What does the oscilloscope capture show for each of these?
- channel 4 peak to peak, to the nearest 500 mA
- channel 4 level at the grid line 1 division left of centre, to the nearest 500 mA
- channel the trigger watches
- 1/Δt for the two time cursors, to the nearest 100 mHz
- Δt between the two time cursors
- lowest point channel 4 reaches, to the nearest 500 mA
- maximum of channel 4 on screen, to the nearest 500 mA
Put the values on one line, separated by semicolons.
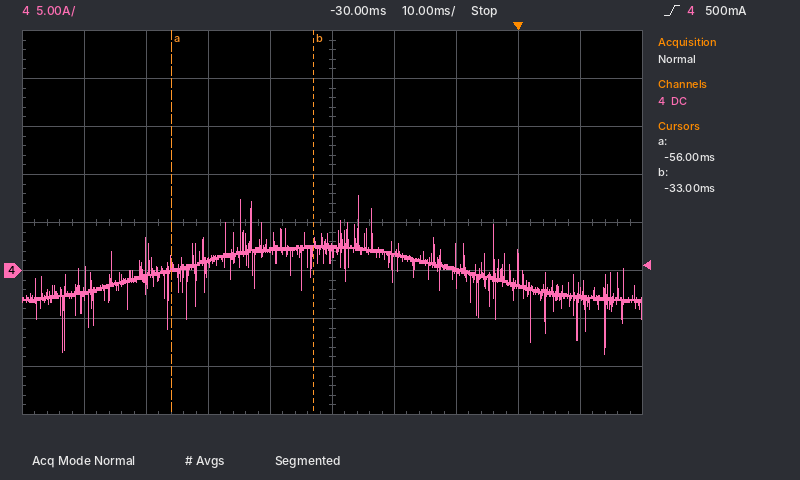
16.5 A; 2.0 A; channel 4; 43.5 Hz; 23 ms; -8.5 A; 8.0 A
